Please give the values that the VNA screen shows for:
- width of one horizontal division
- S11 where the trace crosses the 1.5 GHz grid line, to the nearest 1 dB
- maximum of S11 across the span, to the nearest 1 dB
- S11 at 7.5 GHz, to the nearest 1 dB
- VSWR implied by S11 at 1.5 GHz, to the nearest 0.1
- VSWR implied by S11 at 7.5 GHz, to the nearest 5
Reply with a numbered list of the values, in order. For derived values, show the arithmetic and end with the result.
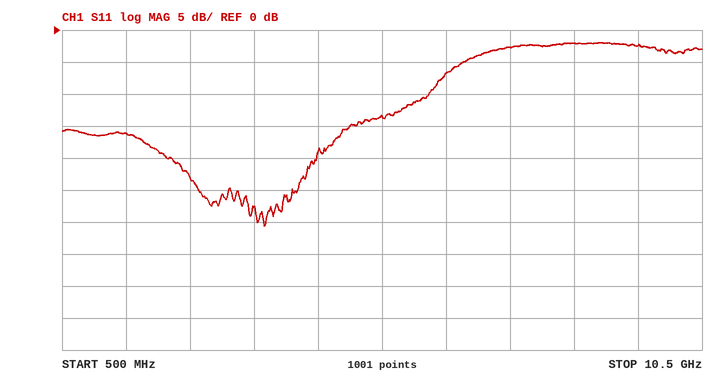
1. 1 GHz
2. -16 dB
3. -2 dB
4. -3 dB
5. |Γ| = 10^(-16/20) = 0.1585; VSWR = (1 + 0.1585)/(1 − 0.1585) ≈ 1.4
6. |Γ| = 10^(-3/20) = 0.7079; VSWR = (1 + 0.7079)/(1 − 0.7079) ≈ 5.85, so 5 to the nearest 5
